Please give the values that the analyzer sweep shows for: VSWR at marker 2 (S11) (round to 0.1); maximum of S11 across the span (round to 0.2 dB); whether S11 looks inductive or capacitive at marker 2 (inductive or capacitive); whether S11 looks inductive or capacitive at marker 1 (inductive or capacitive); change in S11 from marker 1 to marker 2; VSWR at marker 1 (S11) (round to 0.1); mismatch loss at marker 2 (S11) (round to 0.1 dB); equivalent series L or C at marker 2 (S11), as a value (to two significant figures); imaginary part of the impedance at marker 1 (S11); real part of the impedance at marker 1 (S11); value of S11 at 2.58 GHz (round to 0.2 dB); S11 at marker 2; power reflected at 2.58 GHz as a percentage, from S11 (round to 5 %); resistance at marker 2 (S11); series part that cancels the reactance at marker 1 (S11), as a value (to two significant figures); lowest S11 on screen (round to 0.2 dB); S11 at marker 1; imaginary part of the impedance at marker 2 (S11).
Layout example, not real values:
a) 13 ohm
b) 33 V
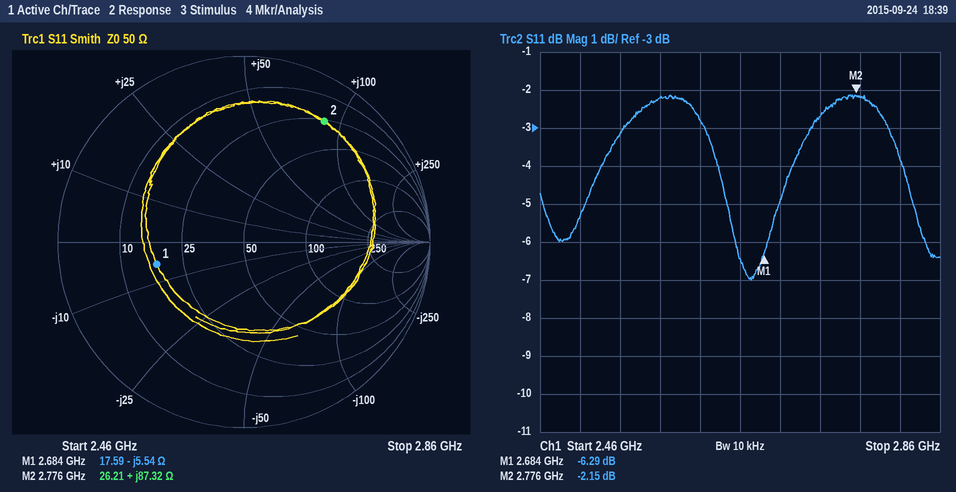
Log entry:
a) 8.1
b) -2.2 dB
c) inductive
d) capacitive
e) 4.14 dB
f) 2.9
g) 4.1 dB
h) 5.0 nH
i) -5.54 Ω
j) 17.59 Ω
k) -2.2 dB
l) -2.15 dB
m) 60 %
n) 26.21 Ω
o) 330 pH
p) -7.0 dB
q) -6.29 dB
r) +87.32 Ω
